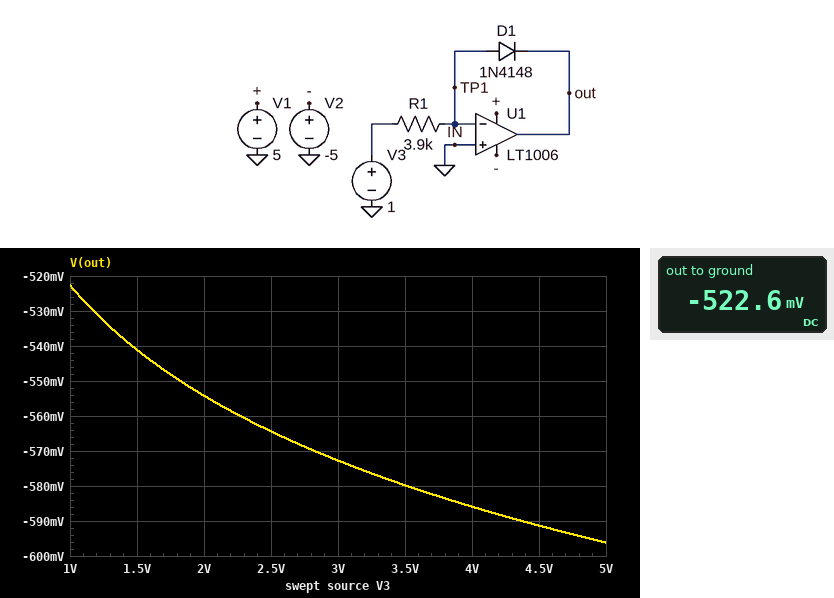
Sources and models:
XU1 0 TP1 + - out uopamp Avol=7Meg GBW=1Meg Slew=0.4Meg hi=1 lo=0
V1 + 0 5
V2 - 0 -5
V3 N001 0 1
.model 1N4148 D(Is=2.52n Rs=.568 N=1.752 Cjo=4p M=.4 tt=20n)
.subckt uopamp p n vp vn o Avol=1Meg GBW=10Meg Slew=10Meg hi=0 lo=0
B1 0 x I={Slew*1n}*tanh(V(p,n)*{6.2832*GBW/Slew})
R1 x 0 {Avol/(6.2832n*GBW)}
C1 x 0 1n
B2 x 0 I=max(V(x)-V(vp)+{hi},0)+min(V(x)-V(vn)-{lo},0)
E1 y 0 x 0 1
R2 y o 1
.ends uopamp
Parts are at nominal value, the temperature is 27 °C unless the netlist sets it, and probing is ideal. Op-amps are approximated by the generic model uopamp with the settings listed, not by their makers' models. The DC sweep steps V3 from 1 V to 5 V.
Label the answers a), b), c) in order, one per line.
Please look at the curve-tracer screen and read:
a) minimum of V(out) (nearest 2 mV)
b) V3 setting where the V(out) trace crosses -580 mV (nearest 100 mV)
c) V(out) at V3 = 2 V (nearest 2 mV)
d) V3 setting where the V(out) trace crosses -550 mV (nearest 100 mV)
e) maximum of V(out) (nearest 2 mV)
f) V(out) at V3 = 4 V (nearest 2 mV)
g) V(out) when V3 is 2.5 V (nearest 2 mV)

a) -596 mV
b) 3.5 V
c) -554 mV
d) 1.8 V
e) -522 mV
f) -586 mV
g) -564 mV
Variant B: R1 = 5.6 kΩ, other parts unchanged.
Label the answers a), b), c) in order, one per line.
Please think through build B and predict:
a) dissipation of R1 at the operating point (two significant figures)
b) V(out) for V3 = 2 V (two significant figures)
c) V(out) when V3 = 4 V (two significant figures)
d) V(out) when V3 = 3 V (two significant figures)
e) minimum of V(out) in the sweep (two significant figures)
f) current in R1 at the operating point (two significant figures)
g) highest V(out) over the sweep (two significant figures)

a) 180 µW
b) -540 mV
c) -570 mV
d) -560 mV
e) -580 mV
f) 180 µA
g) -510 mV
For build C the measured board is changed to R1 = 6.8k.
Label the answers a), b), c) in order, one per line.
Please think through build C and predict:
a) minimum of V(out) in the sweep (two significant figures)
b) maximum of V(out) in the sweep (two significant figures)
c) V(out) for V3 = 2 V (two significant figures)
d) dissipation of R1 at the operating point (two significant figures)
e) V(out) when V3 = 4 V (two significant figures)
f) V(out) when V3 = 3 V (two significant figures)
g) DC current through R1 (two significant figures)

a) -570 mV
b) -500 mV
c) -530 mV
d) 150 µW
e) -560 mV
f) -550 mV
g) 150 µA
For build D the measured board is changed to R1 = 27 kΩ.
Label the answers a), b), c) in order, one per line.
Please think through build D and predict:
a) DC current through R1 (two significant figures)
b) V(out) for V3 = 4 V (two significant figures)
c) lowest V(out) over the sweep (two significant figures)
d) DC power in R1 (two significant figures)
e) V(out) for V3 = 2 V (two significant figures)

a) 37 µA
b) -500 mV
c) -510 mV
d) 37 µW
e) -470 mV
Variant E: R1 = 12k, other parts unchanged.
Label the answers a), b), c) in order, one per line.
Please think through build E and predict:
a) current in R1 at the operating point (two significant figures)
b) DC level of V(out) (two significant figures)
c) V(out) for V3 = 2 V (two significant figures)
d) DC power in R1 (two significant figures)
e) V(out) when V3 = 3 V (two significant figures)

a) 83 µA
b) -470 mV
c) -500 mV
d) 83 µW
e) -520 mV
